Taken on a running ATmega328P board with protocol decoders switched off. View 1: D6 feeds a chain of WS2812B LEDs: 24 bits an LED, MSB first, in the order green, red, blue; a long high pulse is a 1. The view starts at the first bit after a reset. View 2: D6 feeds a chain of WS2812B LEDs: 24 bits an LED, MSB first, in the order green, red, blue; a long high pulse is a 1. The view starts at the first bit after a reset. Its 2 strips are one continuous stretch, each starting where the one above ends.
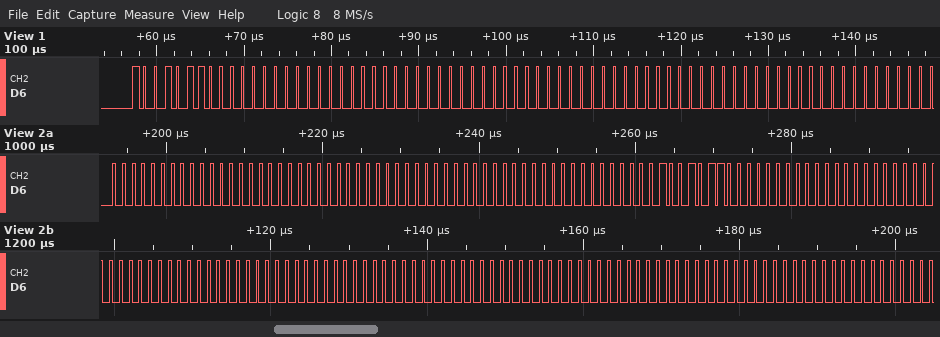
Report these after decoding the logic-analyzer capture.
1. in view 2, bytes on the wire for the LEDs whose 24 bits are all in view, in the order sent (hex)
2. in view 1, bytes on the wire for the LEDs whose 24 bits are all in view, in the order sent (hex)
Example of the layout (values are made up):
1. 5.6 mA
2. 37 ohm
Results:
1. 00 00 00 00 00 00 00 96 00 00 00 00 00 00 00 00 00 00 00 00 00
2. 96 00 00 00 00 00 00 00 00
